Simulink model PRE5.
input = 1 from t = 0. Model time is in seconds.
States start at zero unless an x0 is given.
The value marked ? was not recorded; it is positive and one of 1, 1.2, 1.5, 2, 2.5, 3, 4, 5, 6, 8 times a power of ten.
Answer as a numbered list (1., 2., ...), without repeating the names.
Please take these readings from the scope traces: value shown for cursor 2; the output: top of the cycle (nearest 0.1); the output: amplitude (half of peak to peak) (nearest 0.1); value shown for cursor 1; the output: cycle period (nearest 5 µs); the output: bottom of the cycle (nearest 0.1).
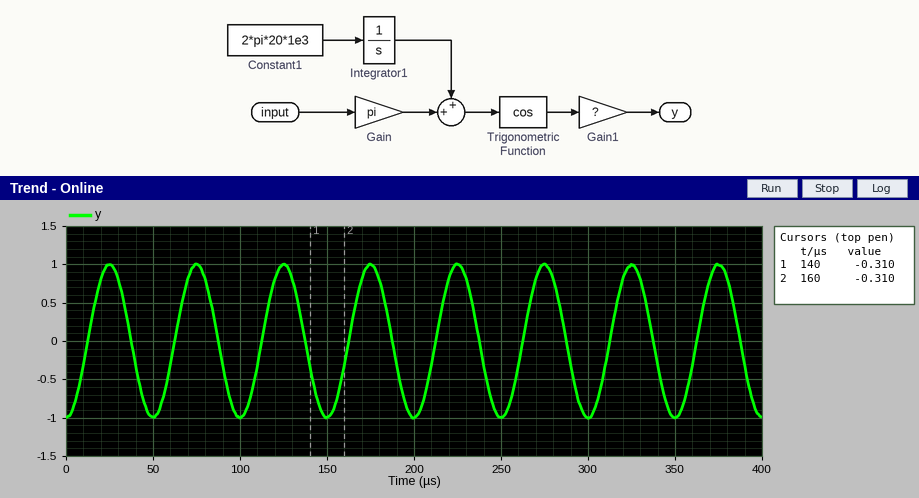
1. -0.310
2. 1.0
3. 1.0
4. -0.310
5. 50 µs
6. -1.0
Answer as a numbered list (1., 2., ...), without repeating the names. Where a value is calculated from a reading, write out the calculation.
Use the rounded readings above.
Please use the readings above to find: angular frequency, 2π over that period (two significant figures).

1. 2π / 50 = 0.13 rad/µs
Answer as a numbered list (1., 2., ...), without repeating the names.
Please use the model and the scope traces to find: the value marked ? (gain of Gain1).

1. 1
